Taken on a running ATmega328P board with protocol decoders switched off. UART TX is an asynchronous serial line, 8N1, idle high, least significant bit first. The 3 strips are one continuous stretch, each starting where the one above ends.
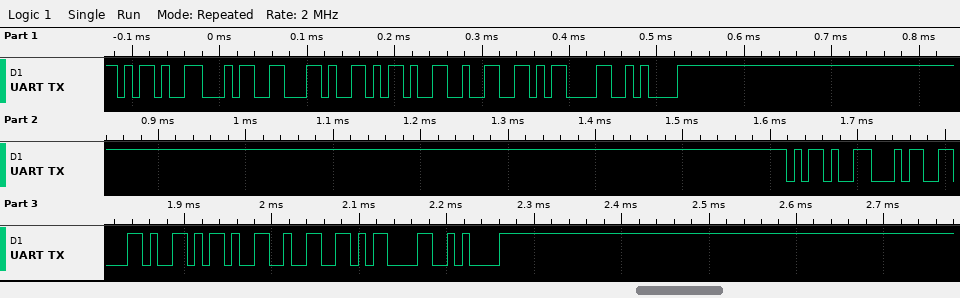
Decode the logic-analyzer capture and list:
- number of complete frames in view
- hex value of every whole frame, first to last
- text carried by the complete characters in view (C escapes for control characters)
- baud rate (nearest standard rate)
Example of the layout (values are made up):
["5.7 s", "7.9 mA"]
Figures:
["14", "0x2D 0x34 0x2C 0x2D 0x32 0x0D 0x0A 0x2D 0x34 0x2C 0x2D 0x32 0x0D 0x0A", "\"-4,-2\\r\\n-4,-2\\r\\n\"", "115200 baud"]
